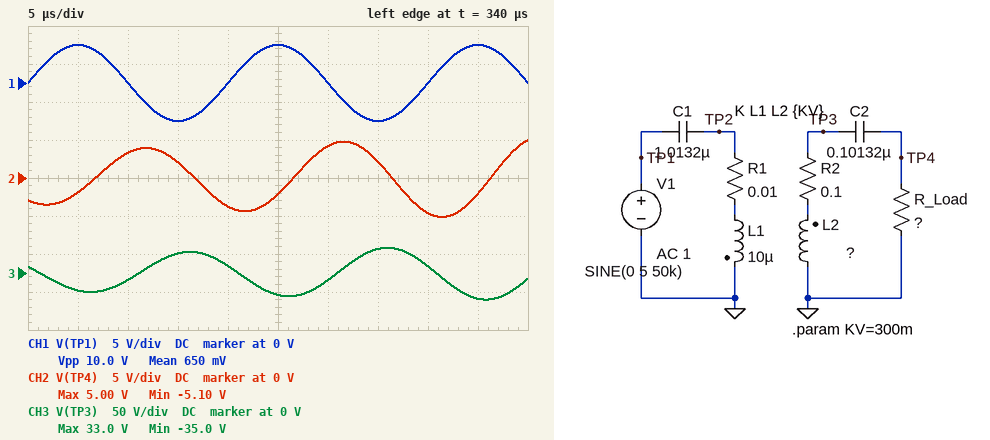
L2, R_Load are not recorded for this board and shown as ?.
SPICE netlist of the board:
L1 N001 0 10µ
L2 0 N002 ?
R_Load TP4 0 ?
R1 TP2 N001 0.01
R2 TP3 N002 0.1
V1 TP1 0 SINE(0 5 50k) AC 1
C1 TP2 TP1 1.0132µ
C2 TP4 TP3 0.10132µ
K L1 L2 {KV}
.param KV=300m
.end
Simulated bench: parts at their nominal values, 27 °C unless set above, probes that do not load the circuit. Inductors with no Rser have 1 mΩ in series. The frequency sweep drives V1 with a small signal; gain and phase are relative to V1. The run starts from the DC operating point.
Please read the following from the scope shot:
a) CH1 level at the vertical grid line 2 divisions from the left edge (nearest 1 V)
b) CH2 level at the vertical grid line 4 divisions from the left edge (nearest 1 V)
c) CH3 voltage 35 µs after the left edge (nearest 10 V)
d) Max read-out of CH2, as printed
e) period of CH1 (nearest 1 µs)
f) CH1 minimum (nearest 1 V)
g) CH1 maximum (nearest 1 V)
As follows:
0 V
-4 V
30 V
5.00 V
20 µs
-5 V
5 V
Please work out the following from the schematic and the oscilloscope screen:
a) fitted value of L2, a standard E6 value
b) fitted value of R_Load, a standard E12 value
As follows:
330 µH
4.7 Ω
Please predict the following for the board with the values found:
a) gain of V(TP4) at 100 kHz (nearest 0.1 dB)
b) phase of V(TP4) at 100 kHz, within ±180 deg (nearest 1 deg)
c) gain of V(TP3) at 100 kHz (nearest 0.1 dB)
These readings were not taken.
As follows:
-23.8 dB
92 deg
-12.9 dB
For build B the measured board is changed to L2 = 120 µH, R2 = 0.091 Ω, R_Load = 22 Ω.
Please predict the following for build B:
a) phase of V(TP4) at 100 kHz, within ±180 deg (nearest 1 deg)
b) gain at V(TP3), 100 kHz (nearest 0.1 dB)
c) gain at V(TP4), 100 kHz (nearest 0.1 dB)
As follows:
114 deg
-3.4 dB
-5.2 dB
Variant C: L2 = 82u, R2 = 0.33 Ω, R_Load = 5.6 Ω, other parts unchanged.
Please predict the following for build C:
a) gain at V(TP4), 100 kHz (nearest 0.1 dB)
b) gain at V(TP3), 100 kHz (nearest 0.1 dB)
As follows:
-13.5 dB
-4.0 dB
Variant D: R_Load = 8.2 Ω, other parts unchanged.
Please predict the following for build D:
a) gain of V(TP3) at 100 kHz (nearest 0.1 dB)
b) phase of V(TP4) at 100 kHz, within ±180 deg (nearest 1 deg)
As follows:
-12.3 dB
93 deg
